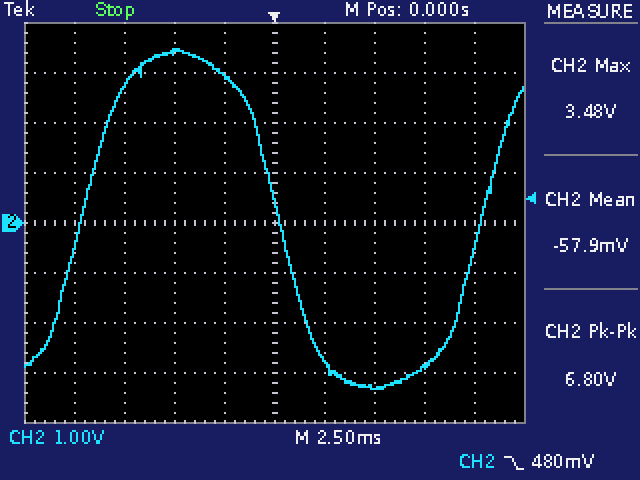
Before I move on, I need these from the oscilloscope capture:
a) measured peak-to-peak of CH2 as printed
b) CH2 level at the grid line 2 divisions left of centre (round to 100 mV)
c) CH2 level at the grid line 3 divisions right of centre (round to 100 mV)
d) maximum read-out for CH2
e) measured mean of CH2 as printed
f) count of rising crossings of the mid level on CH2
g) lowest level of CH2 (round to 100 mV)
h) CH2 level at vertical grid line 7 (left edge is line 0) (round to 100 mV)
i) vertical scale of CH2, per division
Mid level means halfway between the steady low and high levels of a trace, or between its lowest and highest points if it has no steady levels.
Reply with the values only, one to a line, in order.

6.80 V
3.4 V
-2.9 V
3.48 V
-57.9 mV
2
-3.3 V
-3.3 V
1 V
